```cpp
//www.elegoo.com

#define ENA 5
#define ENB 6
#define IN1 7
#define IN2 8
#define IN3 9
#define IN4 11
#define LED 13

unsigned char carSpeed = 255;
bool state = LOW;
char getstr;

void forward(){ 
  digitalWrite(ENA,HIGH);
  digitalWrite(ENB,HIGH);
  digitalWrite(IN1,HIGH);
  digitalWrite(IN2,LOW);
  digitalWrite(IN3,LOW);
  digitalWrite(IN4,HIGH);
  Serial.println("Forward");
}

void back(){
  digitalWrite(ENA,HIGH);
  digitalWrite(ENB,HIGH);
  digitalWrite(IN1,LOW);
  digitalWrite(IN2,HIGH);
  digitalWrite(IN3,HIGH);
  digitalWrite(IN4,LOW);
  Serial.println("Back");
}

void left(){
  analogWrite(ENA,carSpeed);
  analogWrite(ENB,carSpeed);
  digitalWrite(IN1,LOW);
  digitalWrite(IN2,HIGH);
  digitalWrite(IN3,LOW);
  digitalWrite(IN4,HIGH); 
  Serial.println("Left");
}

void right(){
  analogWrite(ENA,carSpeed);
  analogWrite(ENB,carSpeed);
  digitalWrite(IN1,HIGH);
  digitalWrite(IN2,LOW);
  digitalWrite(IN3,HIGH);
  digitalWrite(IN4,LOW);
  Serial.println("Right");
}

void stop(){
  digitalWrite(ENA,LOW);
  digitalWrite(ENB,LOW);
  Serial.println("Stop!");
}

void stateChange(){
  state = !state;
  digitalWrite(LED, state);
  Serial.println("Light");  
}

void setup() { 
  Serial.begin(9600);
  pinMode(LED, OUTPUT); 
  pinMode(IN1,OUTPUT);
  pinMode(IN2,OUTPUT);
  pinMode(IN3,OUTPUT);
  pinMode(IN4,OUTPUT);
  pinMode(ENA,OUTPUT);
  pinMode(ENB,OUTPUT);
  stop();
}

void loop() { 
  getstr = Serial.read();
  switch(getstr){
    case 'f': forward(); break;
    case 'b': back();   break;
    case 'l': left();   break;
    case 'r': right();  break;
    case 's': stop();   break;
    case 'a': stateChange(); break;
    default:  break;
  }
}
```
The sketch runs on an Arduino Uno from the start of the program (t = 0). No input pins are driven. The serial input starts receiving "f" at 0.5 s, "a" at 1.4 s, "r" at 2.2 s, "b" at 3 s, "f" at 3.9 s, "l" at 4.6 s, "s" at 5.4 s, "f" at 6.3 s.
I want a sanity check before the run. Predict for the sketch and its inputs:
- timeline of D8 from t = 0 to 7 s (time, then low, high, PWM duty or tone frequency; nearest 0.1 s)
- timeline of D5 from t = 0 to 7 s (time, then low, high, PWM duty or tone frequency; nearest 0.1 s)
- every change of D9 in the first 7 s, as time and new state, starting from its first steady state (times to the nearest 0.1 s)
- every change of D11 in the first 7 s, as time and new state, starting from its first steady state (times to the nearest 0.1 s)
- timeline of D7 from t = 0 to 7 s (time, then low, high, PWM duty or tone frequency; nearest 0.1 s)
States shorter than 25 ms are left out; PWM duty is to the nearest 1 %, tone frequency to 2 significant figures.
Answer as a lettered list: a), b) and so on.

a) 0 s low; 3 s high; 3.9 s low; 4.6 s high; 6.3 s low
b) 0 s low; 0.5 s high; 5.4 s low; 6.3 s high
c) 0 s low; 2.2 s high; 3.9 s low
d) 0 s low; 0.5 s high; 2.2 s low; 3.9 s high
e) 0 s low; 0.5 s high; 3 s low; 3.9 s high; 4.6 s low; 6.3 s high
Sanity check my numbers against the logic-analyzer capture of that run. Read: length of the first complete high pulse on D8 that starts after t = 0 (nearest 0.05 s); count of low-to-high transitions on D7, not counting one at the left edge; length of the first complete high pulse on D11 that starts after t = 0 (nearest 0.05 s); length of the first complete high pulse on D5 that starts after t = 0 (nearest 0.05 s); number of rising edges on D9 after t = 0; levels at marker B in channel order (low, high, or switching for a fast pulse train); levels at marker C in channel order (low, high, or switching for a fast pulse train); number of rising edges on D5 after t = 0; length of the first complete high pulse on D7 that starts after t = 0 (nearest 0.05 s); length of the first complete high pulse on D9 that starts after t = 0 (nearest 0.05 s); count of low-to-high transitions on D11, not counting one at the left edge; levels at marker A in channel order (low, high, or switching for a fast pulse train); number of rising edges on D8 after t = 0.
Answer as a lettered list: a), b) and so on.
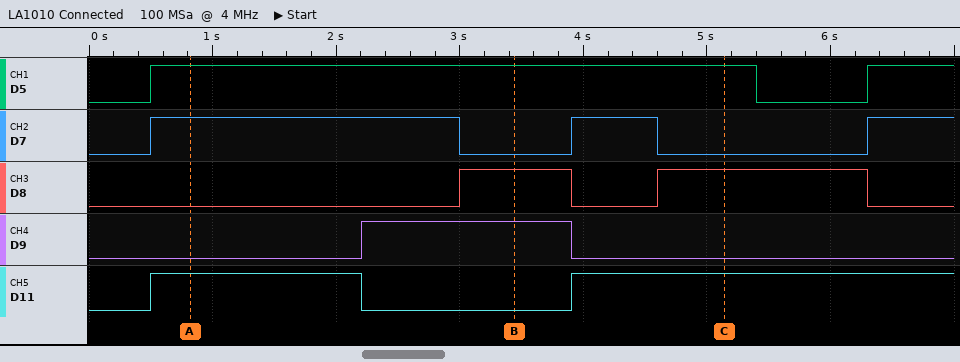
a) 0.90 s
b) 3
c) 1.70 s
d) 4.90 s
e) 1
f) D5 high, D7 low, D8 high, D9 high, D11 low
g) D5 high, D7 low, D8 high, D9 low, D11 high
h) 2
i) 2.50 s
j) 1.70 s
k) 2
l) D5 high, D7 high, D8 low, D9 low, D11 high
m) 2
